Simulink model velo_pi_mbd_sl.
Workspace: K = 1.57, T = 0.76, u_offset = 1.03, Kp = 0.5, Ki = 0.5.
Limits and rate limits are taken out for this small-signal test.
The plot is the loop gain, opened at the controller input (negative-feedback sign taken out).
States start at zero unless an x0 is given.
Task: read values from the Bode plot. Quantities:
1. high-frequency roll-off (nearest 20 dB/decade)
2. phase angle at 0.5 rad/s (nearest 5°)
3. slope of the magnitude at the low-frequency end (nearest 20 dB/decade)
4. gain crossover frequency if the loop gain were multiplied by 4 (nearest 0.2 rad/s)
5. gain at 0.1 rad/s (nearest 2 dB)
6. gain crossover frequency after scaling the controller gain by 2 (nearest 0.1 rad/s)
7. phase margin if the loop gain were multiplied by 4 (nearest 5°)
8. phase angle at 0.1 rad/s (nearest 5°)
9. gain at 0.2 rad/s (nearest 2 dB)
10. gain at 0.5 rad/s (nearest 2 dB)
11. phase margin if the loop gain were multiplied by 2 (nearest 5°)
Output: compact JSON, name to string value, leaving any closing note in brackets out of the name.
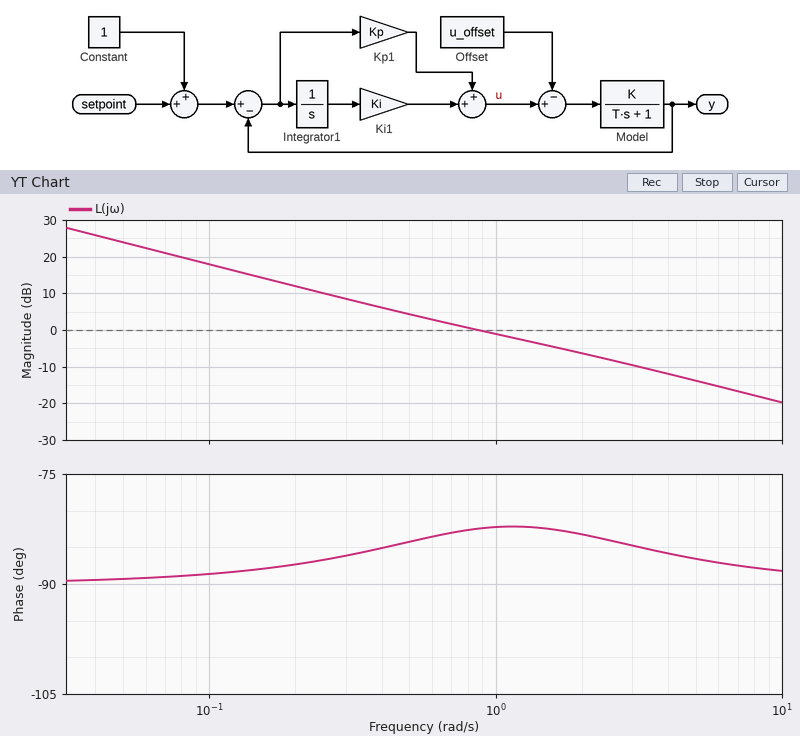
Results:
{"high-frequency roll-off": "-20 dB/decade", "phase angle at 0.5 rad/s": "-85°", "slope of the magnitude at the low-frequency end": "-20 dB/decade", "gain crossover frequency if the loop gain were multiplied by 4": "4.0 rad/s", "gain at 0.1 rad/s": "18 dB", "gain crossover frequency after scaling the controller gain by 2": "1.9 rad/s", "phase margin if the loop gain were multiplied by 4": "95°", "phase angle at 0.1 rad/s": "-90°", "gain at 0.2 rad/s": "12 dB", "gain at 0.5 rad/s": "4 dB", "phase margin if the loop gain were multiplied by 2": "95°"}
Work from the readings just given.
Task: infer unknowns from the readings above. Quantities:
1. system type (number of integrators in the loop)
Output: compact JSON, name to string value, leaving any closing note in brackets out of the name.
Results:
{"system type": "1"}
